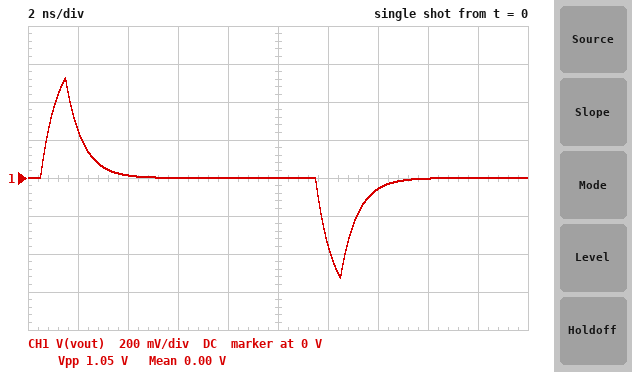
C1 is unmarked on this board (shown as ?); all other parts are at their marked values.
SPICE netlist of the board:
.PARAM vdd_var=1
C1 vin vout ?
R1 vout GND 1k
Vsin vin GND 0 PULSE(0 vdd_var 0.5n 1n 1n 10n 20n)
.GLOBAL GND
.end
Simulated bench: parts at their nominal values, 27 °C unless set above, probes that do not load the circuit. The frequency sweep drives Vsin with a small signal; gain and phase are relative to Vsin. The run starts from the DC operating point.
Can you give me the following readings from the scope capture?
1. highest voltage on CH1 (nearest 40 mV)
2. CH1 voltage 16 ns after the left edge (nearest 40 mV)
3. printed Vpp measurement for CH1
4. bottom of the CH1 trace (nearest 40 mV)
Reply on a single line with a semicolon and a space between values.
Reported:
520 mV; 0 V; 1.05 V; -520 mV
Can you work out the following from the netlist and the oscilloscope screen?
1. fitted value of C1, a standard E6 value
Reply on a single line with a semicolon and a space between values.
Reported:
680 fF
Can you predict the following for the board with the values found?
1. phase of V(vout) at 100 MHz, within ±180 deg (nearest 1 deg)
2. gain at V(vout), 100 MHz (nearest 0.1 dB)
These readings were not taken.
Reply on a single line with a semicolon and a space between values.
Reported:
67 deg; -8.1 dB
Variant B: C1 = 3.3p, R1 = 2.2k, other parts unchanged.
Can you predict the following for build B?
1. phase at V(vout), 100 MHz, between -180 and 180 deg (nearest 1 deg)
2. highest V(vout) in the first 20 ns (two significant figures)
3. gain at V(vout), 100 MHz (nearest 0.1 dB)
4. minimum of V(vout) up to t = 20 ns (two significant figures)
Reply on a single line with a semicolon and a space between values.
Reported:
12 deg; 930 mV; -0.2 dB; -730 mV
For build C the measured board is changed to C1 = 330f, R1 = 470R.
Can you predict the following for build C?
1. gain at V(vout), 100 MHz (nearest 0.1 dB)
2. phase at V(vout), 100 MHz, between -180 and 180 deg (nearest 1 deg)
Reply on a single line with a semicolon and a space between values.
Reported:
-20.3 dB; 84 deg
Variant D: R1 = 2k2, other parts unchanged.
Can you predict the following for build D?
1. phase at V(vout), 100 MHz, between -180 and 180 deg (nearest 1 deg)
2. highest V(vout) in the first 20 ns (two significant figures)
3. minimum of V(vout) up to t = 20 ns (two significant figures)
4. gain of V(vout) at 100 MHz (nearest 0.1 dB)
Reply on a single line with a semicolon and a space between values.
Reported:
47 deg; 730 mV; -730 mV; -3.3 dB
